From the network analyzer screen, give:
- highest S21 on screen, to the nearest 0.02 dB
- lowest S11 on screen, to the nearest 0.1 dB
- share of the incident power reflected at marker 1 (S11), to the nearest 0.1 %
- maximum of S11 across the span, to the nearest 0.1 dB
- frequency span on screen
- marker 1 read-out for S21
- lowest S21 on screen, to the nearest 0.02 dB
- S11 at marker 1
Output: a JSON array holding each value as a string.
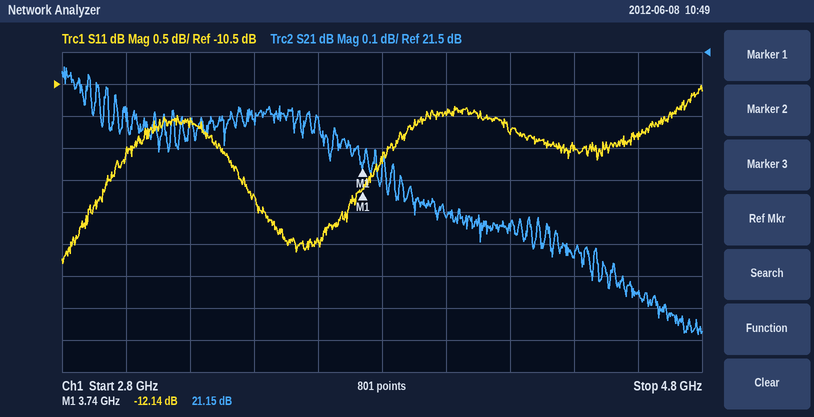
["21.46 dB", "-13.3 dB", "6.1 %", "-10.5 dB", "2 GHz", "21.15 dB", "20.62 dB", "-12.14 dB"]
